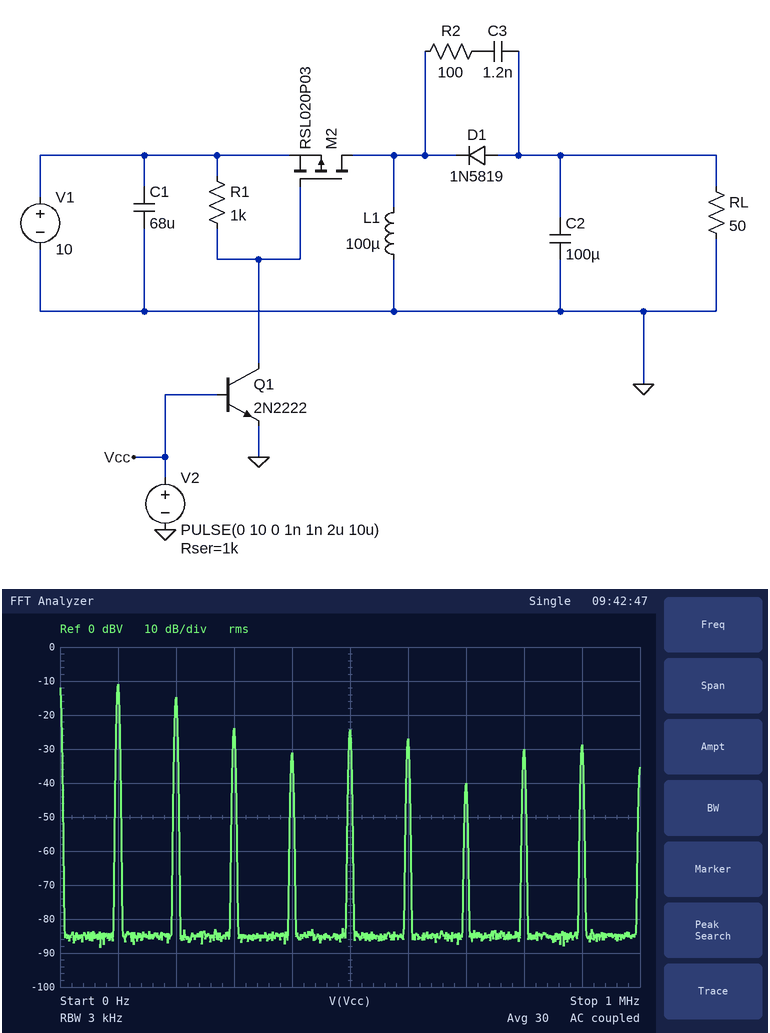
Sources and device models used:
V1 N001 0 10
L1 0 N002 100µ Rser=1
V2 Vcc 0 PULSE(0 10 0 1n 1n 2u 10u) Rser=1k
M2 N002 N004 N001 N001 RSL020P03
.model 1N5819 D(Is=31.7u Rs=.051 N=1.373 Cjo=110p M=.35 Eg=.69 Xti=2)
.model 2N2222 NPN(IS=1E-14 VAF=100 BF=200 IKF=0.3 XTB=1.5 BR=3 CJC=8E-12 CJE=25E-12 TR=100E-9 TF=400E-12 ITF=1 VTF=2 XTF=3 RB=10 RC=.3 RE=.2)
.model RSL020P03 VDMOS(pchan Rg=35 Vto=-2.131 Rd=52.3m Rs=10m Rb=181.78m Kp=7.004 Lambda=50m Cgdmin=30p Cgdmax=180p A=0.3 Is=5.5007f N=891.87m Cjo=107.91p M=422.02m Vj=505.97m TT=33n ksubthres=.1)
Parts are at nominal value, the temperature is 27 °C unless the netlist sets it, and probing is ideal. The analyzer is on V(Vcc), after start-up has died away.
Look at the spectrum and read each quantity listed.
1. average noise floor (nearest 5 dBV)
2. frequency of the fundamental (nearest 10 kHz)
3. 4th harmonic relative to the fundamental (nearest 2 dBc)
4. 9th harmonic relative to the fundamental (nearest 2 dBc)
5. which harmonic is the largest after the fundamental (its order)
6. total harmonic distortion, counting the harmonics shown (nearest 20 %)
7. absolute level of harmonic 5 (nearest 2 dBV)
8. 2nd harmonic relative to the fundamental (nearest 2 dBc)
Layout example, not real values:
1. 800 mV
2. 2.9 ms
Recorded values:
1. -85 dBV
2. 100 kHz
3. -20 dBc
4. -18 dBc
5. 2
6. 80 %
7. -24 dBV
8. -4 dBc
